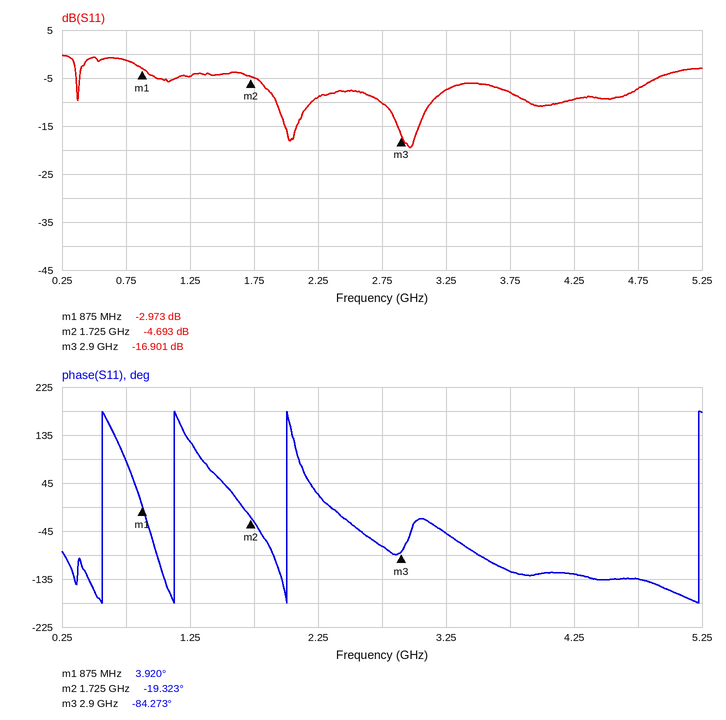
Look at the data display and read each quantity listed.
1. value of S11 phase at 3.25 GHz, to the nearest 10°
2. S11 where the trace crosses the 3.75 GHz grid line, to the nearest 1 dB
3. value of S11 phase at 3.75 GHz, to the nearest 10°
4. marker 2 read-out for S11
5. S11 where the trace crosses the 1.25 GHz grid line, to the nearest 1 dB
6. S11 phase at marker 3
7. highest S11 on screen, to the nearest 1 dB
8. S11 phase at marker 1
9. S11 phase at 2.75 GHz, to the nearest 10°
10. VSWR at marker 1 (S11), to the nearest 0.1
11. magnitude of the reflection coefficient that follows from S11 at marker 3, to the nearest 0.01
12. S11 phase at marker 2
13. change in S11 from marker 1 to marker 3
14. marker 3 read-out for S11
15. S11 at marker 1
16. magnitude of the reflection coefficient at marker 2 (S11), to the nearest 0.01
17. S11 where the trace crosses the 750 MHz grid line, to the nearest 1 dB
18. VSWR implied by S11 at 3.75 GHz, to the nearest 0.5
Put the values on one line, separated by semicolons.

-50°; -8 dB; -120°; -4.693 dB; -5 dB; -84.273°; 0 dB; 3.920°; -70°; 5.9; 0.14; -19.323°; -13.928 dB; -16.901 dB; -2.973 dB; 0.58; -1 dB; 2.5
